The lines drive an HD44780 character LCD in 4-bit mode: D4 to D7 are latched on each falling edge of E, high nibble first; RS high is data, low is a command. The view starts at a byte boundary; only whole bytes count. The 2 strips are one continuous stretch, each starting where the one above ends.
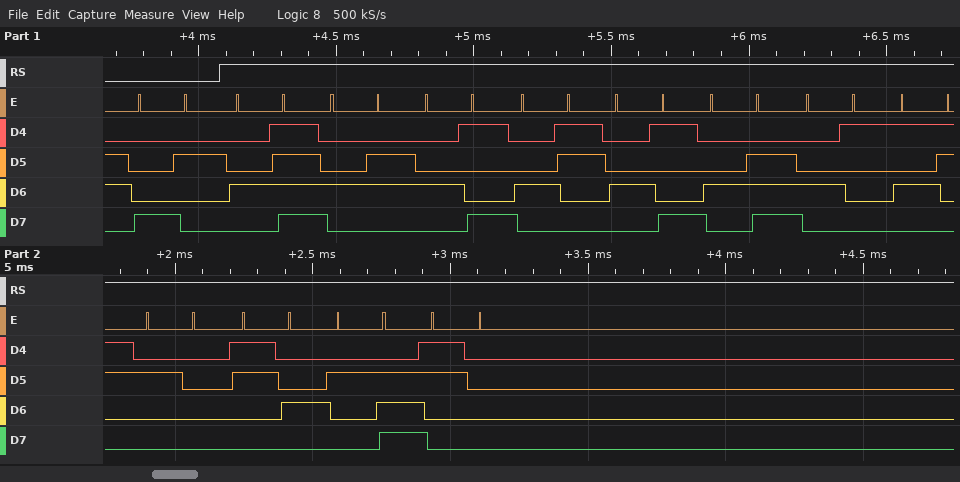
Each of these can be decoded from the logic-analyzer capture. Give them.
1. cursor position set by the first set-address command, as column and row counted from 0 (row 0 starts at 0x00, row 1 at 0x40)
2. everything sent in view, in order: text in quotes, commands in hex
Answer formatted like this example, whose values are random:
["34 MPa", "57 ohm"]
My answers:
["column 2, row 0", "0x82 \"OFICINAS 4.0\""]
